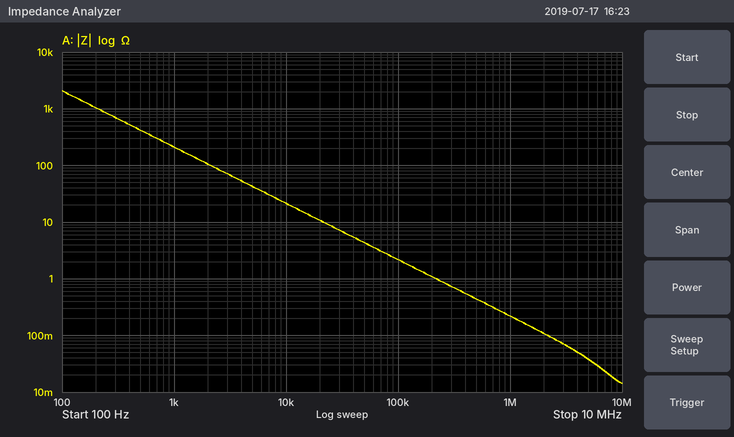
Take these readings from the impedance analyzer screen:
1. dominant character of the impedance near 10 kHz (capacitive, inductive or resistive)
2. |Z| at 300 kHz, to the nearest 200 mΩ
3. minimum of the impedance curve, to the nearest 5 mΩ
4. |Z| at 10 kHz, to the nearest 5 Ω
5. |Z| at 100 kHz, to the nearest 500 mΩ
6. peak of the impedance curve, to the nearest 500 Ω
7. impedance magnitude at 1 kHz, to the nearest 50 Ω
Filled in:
capacitive
800 mΩ
15 mΩ
20 Ω
2.0 Ω
2.0 kΩ
200 Ω
